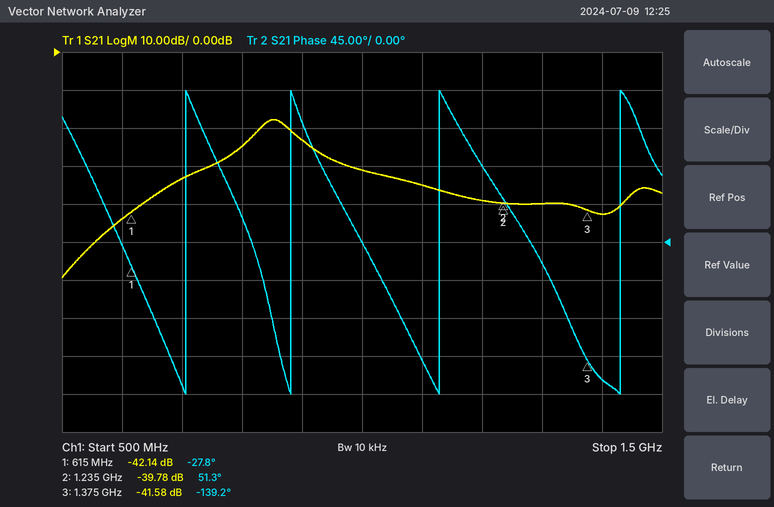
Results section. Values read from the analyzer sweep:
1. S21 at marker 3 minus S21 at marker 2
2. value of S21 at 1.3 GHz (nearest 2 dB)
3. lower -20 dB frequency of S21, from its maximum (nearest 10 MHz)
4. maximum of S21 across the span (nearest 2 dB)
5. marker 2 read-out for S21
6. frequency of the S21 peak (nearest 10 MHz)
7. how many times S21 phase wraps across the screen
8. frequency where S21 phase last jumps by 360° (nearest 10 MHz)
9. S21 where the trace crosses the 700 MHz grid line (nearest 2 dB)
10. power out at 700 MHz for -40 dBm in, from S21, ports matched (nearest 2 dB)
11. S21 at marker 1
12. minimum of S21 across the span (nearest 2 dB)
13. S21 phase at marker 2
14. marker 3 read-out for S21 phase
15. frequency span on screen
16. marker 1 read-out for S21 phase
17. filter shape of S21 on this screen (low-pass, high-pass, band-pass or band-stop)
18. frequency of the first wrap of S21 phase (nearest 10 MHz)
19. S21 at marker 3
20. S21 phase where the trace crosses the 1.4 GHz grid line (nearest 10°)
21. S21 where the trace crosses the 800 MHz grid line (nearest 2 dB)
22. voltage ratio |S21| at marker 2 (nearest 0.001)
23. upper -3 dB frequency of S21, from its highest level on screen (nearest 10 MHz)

-1.80 dB
-40 dB
650 MHz
-18 dB
-39.78 dB
850 MHz
4
1.43 GHz
-34 dB
-74 dBm
-42.14 dB
-60 dB
51.3°
-139.2°
1 GHz
-27.8°
band-pass
710 MHz
-41.58 dB
-160°
-24 dB
0.010
880 MHz
